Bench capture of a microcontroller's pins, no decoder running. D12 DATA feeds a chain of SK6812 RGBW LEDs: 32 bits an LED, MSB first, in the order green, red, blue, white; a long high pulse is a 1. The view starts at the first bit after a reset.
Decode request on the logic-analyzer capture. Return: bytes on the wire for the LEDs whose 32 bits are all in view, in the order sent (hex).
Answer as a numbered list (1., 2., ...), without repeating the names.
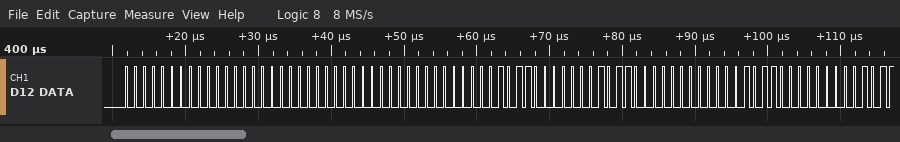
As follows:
1. 00 00 00 00 00 58 0B 00
